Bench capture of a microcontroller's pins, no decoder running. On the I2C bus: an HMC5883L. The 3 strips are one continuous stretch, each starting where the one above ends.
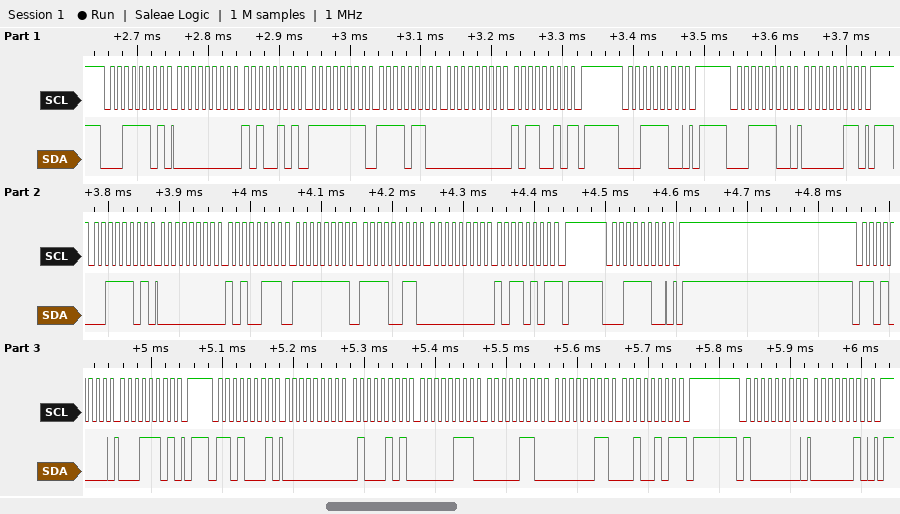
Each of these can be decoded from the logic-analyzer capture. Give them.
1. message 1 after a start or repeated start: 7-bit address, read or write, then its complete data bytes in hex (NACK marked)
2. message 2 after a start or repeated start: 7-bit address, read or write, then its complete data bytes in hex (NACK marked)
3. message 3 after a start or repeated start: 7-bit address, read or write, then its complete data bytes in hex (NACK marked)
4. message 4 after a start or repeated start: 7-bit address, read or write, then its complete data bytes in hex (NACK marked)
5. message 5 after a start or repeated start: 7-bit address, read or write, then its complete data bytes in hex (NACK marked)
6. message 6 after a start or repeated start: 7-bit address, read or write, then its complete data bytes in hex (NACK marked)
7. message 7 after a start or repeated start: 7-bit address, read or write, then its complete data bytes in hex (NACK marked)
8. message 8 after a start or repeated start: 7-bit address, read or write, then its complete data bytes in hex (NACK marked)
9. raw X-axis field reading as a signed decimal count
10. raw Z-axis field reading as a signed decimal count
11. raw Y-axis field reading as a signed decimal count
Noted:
0x1E read: 00 A5 FF F6 00 B2 NACK
0x1E write
0x1E write: 03
0x1E read: 00 A7 FF F3 00 B5 NACK
0x1E write
0x68 write: 1D
0x68 read: 00 45 07 06 03 25 NACK
0x40 write: 02
167
-13
181
